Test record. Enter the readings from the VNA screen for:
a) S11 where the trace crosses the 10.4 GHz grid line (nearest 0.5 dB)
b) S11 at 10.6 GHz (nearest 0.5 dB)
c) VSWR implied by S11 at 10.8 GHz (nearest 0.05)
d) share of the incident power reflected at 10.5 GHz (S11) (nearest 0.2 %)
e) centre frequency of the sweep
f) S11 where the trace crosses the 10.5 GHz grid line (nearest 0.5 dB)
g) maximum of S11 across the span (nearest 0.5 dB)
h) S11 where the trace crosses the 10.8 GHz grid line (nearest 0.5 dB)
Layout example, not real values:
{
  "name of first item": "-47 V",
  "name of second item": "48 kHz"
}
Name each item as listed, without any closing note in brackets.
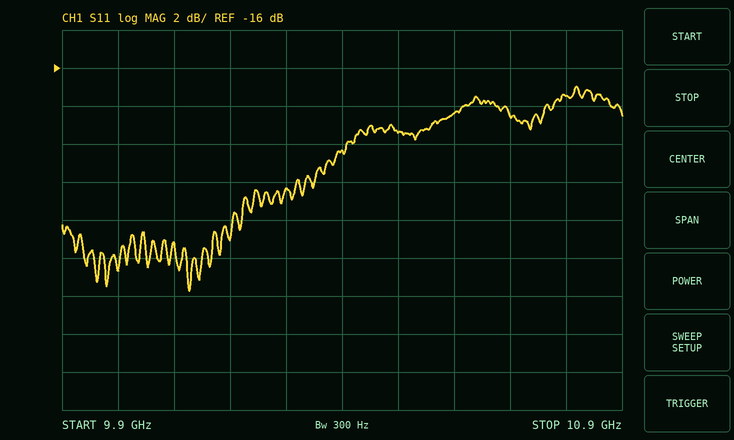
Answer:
{
  "S11 where the trace crosses the 10.4 GHz grid line": "-20.5 dB",
  "S11 at 10.6 GHz": "-18.5 dB",
  "VSWR implied by S11 at 10.8 GHz": "1.30",
  "share of the incident power reflected at 10.5 GHz (S11)": "1.2 %",
  "centre frequency of the sweep": "10.4 GHz",
  "S11 where the trace crosses the 10.5 GHz grid line": "-19.5 dB",
  "maximum of S11 across the span": "-17.0 dB",
  "S11 where the trace crosses the 10.8 GHz grid line": "-17.5 dB"
}
